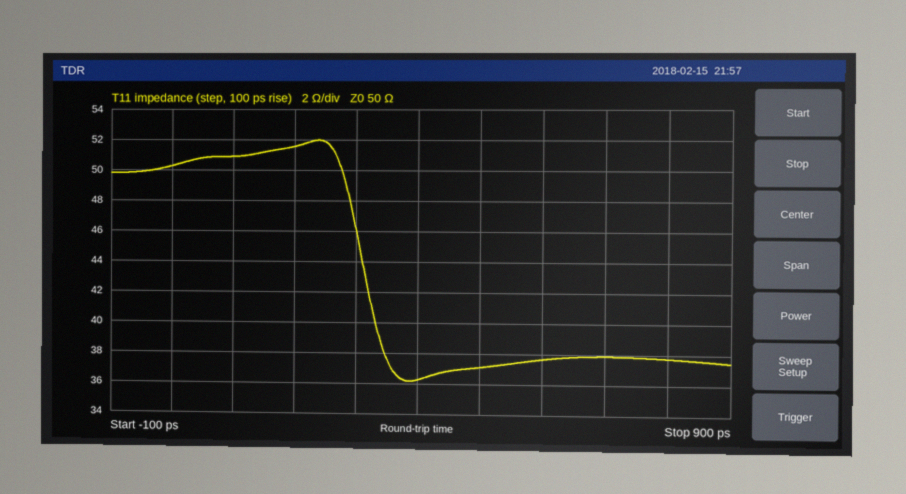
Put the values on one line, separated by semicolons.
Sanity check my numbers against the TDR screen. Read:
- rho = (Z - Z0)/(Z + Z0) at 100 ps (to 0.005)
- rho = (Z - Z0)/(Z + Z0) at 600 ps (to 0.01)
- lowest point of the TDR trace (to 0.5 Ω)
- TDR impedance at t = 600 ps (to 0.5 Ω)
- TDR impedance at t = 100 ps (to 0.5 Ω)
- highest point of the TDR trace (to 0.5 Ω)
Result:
+0.010; -0.14; 36.0 Ω; 37.5 Ω; 51.0 Ω; 52.0 Ω
